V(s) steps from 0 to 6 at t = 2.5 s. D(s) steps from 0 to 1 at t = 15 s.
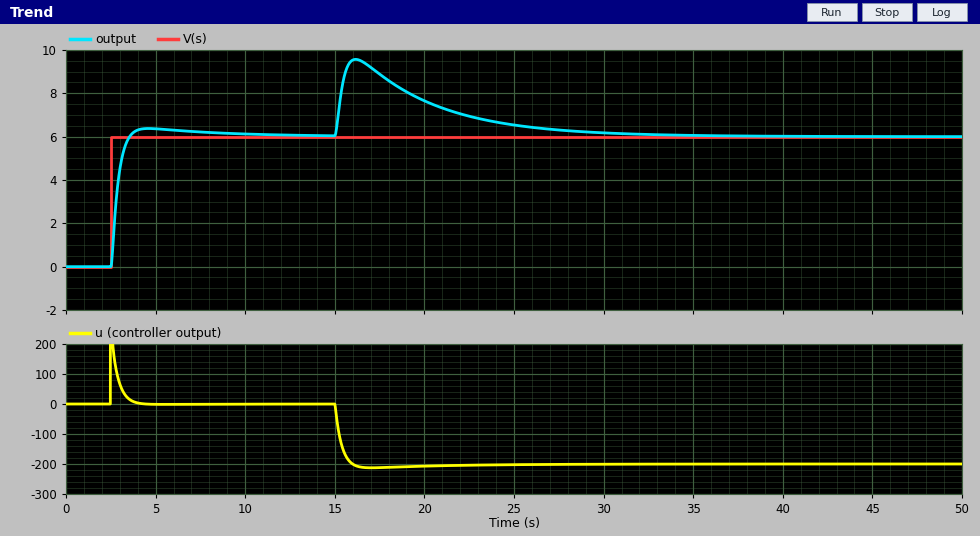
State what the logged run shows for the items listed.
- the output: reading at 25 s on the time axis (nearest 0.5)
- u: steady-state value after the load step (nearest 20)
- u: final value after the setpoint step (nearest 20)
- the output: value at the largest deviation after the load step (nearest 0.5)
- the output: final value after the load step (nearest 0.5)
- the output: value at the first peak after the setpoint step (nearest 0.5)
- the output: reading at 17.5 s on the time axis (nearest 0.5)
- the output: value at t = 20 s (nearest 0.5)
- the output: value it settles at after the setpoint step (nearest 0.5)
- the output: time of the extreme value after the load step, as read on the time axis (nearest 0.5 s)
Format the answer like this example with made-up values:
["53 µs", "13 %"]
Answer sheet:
["6.5", "-200", "0", "9.5", "6.0", "6.5", "9.0", "7.5", "6.0", "16.0 s"]
